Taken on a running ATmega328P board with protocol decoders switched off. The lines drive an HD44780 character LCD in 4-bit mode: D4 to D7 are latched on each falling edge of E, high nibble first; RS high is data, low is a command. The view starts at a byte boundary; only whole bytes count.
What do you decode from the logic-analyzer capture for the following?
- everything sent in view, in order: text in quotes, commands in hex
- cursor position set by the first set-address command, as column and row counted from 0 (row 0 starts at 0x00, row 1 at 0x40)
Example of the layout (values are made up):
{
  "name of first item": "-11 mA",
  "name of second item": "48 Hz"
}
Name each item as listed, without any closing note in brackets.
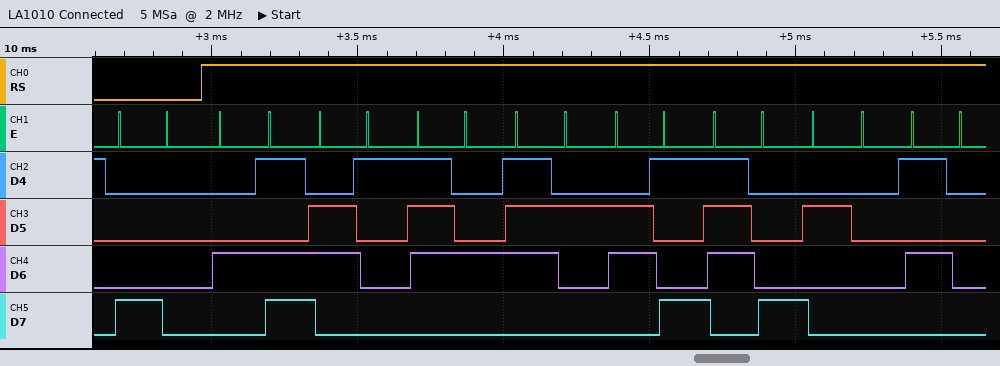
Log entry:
{
  "everything sent in view, in order: text in quotes, commands in hex": "0x80 \"Matrix P\"",
  "cursor position set by the first set-address command, as column and row counted from 0": "column 0, row 0"
}
